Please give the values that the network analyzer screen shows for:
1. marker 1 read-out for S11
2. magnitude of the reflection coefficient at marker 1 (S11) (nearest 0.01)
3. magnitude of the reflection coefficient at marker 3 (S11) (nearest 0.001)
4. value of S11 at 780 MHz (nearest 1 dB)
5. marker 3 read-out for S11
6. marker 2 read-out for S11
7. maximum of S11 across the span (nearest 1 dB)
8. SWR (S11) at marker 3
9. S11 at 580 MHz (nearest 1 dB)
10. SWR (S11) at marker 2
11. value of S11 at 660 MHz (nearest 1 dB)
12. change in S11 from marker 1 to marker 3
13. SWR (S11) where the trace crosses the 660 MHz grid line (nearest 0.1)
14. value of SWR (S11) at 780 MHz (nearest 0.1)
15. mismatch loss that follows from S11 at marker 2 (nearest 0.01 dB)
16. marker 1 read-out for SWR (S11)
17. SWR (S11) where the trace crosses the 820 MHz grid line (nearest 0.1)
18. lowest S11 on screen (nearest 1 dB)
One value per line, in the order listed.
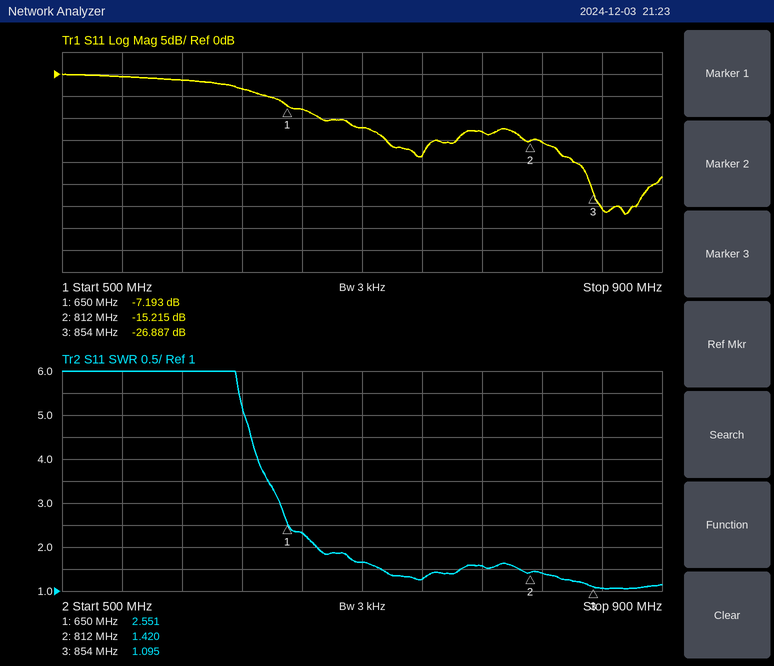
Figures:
-7.193 dB
0.44
0.045
-13 dB
-26.887 dB
-15.215 dB
0 dB
1.095
-1 dB
1.420
-8 dB
-19.694 dB
2.3
1.6
0.13 dB
2.551
1.4
-32 dB
